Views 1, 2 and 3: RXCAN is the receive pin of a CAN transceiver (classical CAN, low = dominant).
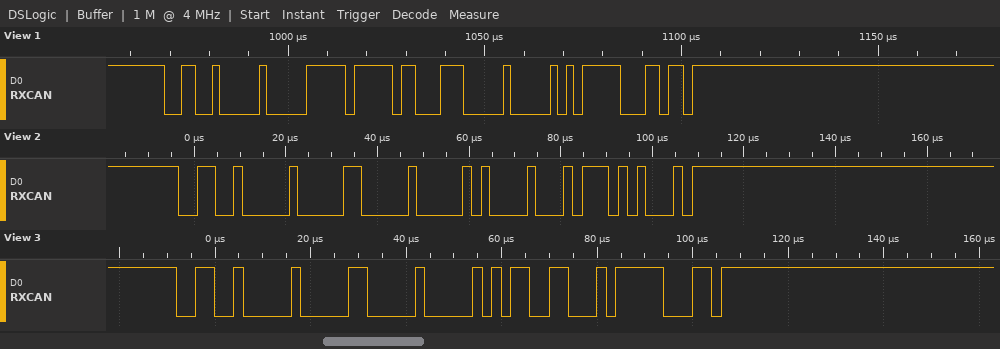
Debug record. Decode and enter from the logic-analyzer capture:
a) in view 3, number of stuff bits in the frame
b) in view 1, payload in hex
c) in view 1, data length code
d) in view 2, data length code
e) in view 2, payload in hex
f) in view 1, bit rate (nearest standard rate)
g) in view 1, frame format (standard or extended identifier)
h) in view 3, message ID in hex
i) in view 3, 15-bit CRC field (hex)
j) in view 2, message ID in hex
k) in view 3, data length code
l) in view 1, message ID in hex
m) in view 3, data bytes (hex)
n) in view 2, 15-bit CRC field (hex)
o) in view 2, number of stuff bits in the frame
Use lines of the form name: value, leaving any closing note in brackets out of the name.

in view 3, number of stuff bits in the frame: 5
in view 1, payload in hex: FF 8E 00
in view 1, data length code: 3
in view 2, data length code: 2
in view 2, payload in hex: 00 21
in view 1, bit rate: 500 kbit/s
in view 1, frame format: standard
in view 3, message ID in hex: 0x320
in view 3, 15-bit CRC field: 0x62F9
in view 2, message ID in hex: 0x320
in view 3, data length code: 2
in view 1, message ID in hex: 0x320
in view 3, data bytes: 00 2C
in view 2, 15-bit CRC field: 0x0BA8
in view 2, number of stuff bits in the frame: 4
